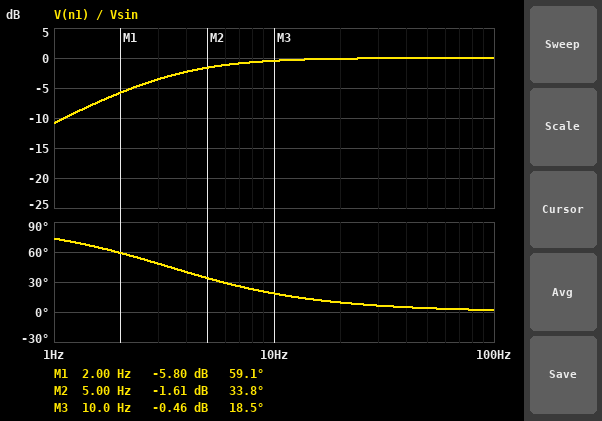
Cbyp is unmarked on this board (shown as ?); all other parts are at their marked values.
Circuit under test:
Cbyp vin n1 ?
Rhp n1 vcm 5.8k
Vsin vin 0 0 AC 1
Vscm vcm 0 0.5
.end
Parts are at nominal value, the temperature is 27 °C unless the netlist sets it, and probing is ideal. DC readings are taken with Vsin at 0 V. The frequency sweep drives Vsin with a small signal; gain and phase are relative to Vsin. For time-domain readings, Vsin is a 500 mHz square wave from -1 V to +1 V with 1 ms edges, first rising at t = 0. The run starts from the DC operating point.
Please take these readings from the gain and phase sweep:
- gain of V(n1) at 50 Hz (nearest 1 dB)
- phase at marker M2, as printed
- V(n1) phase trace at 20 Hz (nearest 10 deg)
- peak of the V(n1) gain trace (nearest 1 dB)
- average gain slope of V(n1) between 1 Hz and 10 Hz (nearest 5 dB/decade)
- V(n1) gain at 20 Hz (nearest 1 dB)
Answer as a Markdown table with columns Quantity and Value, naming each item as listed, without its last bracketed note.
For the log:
| Quantity | Value |
|---|---|
| gain of V(n1) at 50 Hz | 0 dB |
| phase at marker M2, as printed | 33.8 deg |
| V(n1) phase trace at 20 Hz | 10 deg |
| peak of the V(n1) gain trace | 0 dB |
| average gain slope of V(n1) between 1 Hz and 10 Hz | 10 dB/decade |
| V(n1) gain at 20 Hz | 0 dB |
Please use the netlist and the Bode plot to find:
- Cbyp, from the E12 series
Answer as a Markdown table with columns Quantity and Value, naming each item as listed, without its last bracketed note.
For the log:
| Quantity | Value |
|---|---|
| Cbyp, from the E12 series | 8.2 µF |
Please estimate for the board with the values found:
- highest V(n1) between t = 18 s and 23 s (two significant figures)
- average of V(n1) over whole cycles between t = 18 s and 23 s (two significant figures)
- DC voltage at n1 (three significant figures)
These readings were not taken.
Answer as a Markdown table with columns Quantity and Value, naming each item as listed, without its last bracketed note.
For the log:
| Quantity | Value |
|---|---|
| highest V(n1) between t = 18 s and 23 s | 2.5 V |
| average of V(n1) over whole cycles between t = 18 s and 23 s | 500 mV |
| DC voltage at n1 | 500 mV |
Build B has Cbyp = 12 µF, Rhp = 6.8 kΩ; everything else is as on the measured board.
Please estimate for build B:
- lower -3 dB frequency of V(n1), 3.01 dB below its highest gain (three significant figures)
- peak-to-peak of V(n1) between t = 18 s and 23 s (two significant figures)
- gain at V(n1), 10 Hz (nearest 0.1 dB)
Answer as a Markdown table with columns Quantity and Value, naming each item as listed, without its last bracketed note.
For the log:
| Quantity | Value |
|---|---|
| lower -3 dB frequency of V(n1), 3.01 dB below its highest gain | 1.95 Hz |
| peak-to-peak of V(n1) between t = 18 s and 23 s | 4.0 V |
| gain at V(n1), 10 Hz | -0.2 dB |
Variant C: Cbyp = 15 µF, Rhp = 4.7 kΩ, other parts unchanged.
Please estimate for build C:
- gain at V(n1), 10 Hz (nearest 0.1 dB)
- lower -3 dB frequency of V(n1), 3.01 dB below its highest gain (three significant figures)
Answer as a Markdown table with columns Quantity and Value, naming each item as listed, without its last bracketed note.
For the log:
| Quantity | Value |
|---|---|
| gain at V(n1), 10 Hz | -0.2 dB |
| lower -3 dB frequency of V(n1), 3.01 dB below its highest gain | 2.26 Hz |
